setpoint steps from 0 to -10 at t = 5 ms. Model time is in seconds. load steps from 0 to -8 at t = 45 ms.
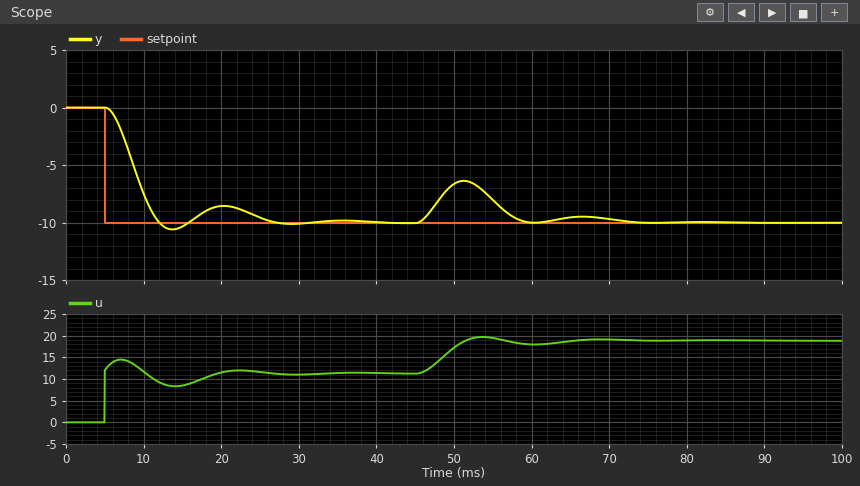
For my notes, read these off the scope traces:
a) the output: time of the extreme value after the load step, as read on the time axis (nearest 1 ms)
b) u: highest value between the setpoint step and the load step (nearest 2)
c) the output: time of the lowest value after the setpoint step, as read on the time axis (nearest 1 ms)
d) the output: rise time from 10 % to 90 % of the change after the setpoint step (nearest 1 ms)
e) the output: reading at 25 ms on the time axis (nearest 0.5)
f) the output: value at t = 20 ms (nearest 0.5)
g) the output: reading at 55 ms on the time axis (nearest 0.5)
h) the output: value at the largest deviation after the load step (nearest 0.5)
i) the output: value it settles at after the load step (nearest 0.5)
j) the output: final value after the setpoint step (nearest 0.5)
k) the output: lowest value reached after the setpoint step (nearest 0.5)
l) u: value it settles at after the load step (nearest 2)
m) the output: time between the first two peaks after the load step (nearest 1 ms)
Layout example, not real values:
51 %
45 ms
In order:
51 ms
14
14 ms
5 ms
-9.5
-8.5
-8.0
-6.5
-10.0
-10.0
-10.5
18
15 ms
